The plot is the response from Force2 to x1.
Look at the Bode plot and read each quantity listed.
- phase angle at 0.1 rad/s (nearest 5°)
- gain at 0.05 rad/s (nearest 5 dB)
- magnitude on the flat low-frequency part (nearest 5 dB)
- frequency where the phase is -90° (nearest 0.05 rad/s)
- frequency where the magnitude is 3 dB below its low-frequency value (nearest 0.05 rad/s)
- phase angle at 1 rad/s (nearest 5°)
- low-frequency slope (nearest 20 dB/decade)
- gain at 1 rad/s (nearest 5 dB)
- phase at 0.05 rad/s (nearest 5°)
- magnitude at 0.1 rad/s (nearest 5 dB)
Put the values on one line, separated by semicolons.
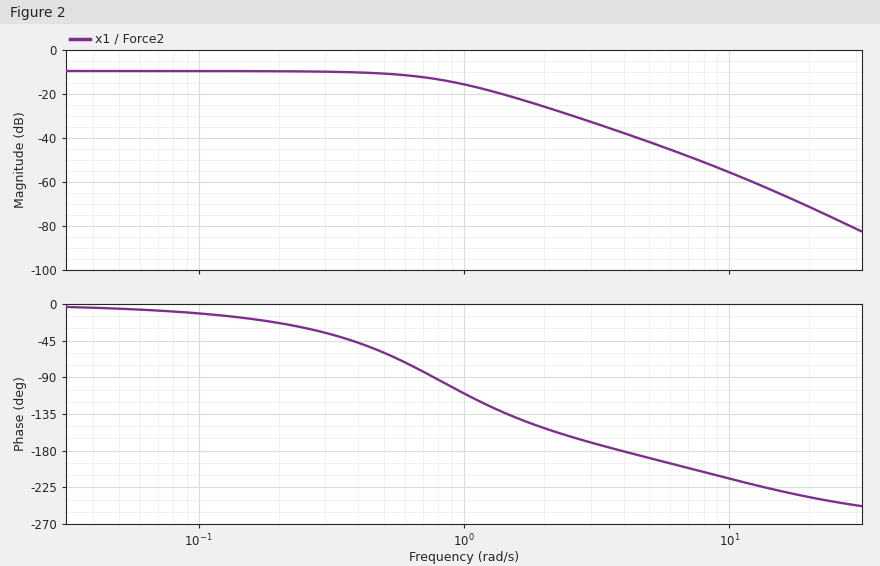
-10°; -10 dB; -10 dB; 0.75 rad/s; 0.70 rad/s; -110°; 0 dB/decade; -15 dB; -5°; -10 dB
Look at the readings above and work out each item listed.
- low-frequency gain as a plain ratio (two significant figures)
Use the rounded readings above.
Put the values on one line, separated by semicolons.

0.32
